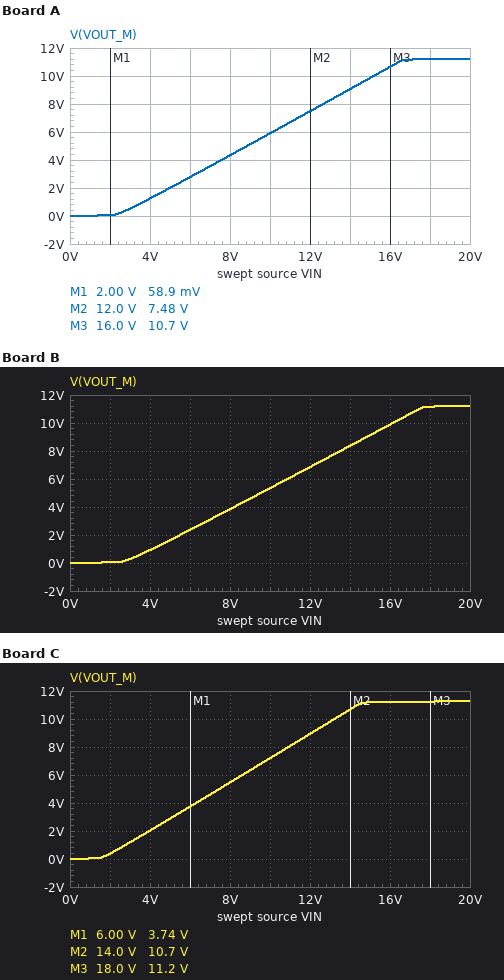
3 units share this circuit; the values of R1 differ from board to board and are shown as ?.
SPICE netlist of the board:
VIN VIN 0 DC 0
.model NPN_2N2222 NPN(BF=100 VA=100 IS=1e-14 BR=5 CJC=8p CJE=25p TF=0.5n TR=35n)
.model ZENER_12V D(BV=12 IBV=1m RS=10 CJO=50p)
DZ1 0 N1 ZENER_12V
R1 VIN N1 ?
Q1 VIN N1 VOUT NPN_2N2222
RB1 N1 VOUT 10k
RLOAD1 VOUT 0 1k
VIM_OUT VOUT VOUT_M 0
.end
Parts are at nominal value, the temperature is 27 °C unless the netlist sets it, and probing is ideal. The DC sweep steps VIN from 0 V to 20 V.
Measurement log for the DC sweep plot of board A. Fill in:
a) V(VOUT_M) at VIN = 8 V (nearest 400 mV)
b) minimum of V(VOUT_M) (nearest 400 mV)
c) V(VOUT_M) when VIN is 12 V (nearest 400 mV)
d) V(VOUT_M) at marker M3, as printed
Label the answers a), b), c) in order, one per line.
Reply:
a) 4.4 V
b) 0 V
c) 7.6 V
d) 10.7 V
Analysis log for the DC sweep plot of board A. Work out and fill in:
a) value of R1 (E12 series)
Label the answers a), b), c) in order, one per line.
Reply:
a) 27 kΩ
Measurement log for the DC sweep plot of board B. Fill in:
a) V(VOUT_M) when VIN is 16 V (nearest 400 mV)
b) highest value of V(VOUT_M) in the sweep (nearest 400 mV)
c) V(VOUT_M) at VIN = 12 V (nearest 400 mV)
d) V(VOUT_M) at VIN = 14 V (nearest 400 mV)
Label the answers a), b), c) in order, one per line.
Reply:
a) 10.0 V
b) 11.2 V
c) 6.8 V
d) 8.4 V
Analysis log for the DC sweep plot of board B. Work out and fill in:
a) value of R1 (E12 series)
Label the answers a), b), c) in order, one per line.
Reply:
a) 33 kΩ
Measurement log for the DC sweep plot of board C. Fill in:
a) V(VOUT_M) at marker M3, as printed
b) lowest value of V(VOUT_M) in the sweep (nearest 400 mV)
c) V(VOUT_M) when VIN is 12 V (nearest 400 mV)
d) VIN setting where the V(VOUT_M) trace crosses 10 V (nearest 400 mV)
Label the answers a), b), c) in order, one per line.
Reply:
a) 11.2 V
b) 0 V
c) 8.8 V
d) 13.2 V
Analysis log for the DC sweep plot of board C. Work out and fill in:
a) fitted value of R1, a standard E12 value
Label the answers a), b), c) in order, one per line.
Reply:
a) 15 kΩ
